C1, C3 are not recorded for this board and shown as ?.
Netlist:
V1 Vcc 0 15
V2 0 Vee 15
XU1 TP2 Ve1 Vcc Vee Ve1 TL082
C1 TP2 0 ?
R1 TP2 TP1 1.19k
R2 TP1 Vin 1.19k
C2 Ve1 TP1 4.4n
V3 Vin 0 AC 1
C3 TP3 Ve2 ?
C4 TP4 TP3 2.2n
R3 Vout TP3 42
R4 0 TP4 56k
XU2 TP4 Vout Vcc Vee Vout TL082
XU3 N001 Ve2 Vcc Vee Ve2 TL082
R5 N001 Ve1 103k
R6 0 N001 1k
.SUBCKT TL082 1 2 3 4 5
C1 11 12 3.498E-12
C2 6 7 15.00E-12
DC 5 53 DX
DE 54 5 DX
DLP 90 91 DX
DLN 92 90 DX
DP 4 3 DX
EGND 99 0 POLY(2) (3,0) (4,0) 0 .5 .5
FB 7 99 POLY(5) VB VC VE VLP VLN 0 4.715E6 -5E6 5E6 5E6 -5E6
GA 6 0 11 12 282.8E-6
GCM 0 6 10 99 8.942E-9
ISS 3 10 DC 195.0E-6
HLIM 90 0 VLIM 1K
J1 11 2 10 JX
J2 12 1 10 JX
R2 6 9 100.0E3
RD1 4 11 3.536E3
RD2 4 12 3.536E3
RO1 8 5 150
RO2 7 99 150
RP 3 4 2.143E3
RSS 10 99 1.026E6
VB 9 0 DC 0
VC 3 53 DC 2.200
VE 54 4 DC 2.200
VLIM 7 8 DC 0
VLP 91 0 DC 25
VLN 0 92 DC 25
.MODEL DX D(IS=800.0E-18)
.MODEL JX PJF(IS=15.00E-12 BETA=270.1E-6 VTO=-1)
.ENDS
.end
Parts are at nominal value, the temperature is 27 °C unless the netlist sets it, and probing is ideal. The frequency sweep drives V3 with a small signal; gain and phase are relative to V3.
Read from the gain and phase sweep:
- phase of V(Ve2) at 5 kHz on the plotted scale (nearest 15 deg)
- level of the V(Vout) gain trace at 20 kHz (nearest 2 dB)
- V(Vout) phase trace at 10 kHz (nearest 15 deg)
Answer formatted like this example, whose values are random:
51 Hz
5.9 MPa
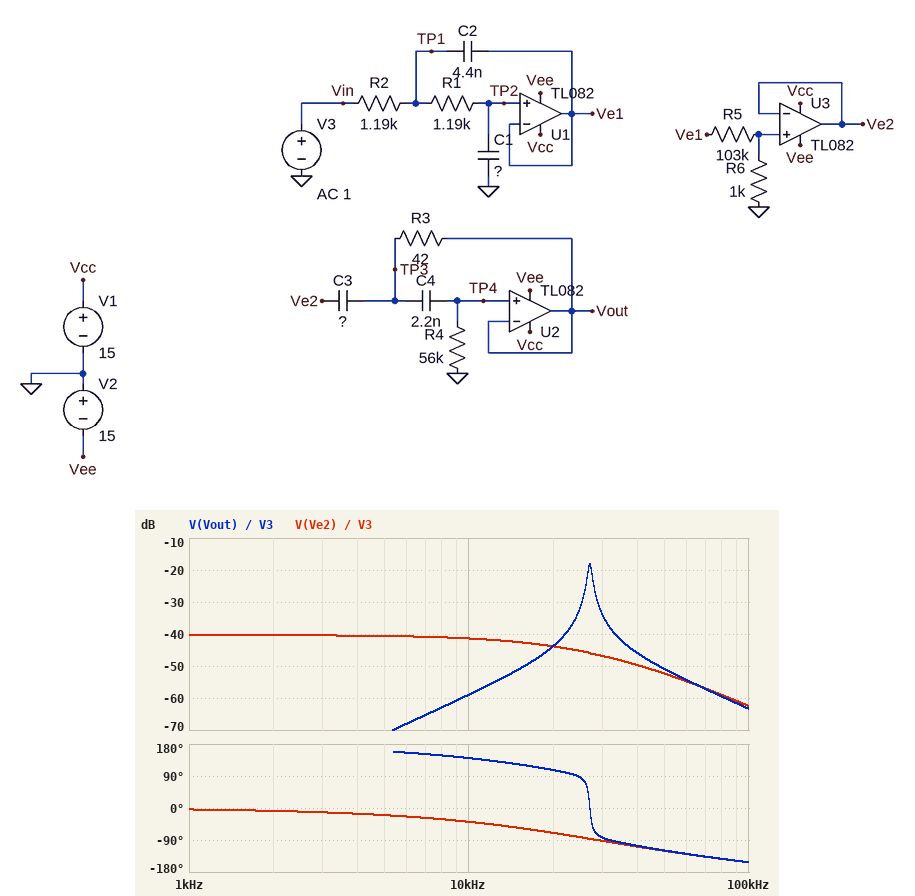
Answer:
-15 deg
-44 dB
135 deg
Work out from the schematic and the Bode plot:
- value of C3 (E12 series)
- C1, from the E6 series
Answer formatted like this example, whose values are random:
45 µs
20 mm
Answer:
5.6 nF
4.7 nF
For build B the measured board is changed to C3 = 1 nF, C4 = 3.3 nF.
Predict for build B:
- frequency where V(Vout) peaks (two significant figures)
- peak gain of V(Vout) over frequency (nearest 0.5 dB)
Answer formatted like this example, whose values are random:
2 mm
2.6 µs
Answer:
39 kHz
-25.5 dB
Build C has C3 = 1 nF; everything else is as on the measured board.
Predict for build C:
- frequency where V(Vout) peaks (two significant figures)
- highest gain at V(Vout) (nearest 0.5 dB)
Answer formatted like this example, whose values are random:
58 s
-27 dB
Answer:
48 kHz
-25.0 dB
